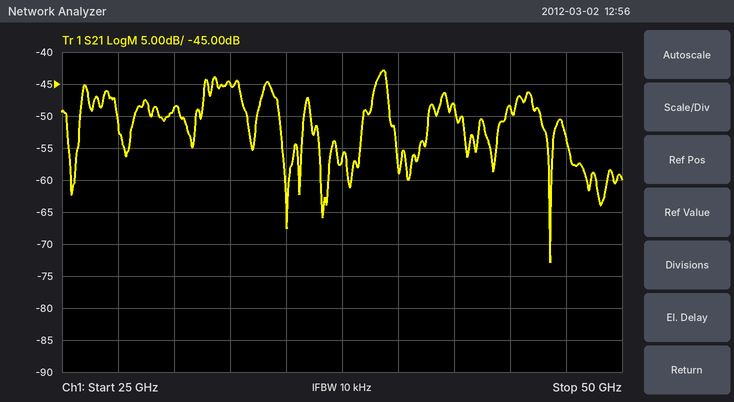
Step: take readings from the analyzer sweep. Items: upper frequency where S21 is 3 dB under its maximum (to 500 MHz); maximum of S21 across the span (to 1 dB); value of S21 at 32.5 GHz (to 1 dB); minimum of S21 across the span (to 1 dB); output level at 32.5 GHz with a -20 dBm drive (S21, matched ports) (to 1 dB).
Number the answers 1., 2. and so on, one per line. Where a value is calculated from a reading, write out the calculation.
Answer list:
1. 39.5 GHz
2. -43 dB
3. -45 dB
4. -73 dB
5. -20 dBm + (-45 dB) = -65 dBm
